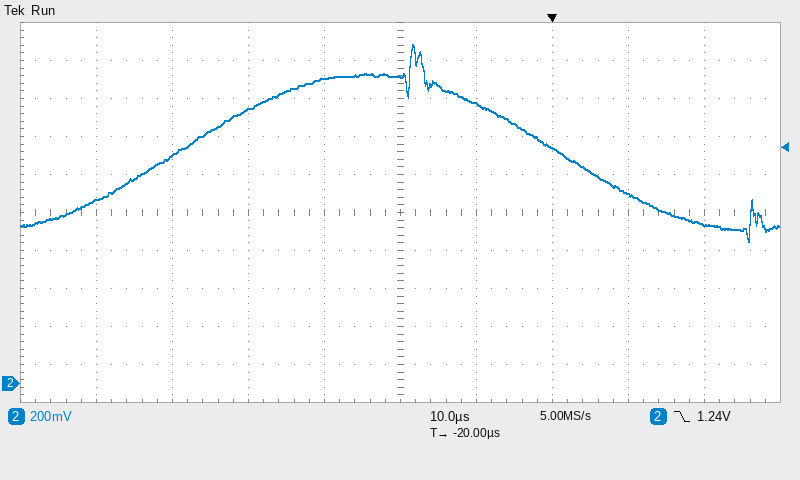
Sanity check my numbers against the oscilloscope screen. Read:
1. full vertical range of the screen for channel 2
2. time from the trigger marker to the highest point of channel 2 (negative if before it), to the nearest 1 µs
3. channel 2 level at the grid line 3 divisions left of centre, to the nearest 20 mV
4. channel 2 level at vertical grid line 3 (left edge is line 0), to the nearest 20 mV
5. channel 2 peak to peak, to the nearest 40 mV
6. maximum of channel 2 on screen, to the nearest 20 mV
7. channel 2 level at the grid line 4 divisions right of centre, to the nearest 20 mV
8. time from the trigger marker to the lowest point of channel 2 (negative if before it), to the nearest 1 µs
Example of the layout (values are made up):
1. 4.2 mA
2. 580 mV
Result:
1. 2 V
2. -18 µs
3. 1.20 V
4. 1.44 V
5. 1.04 V
6. 1.78 V
7. 840 mV
8. +26 µs
